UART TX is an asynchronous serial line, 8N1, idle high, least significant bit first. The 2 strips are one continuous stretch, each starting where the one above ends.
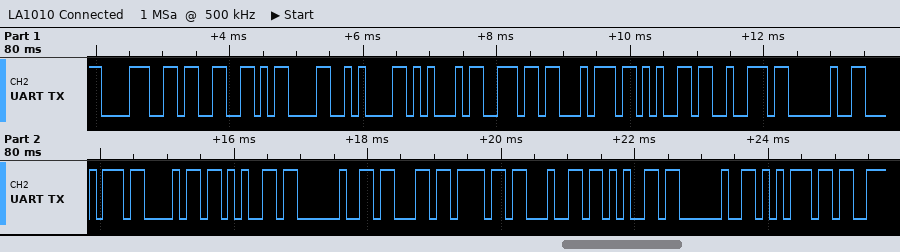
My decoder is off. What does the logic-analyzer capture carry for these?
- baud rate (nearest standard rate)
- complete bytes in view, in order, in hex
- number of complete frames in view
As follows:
9600 baud
38 33 0D 0A 45 6E 74 65 72 20 74 68 65 20 63 6F 64 65 20 75
20
